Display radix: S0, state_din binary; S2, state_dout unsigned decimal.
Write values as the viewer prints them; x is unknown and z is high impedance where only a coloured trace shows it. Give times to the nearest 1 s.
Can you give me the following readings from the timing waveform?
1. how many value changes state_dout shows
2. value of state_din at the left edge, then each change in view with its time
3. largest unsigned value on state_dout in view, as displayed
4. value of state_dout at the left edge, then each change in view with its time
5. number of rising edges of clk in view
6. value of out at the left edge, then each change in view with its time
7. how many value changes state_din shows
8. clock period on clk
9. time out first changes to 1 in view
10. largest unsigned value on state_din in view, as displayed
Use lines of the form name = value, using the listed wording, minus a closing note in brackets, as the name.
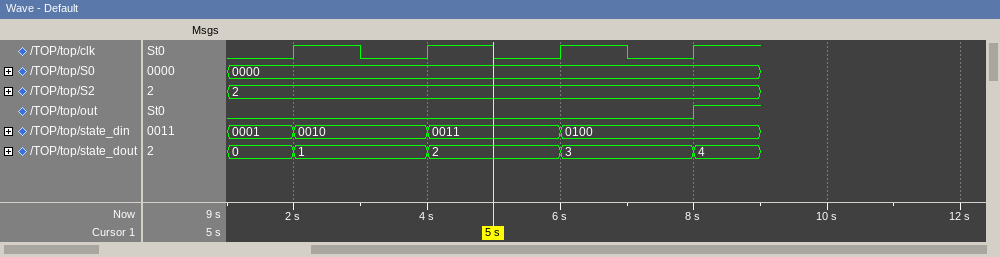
how many value changes state_dout shows = 4
value of state_din at the left edge, then each change in view with its time = 0001, 0010 at 2 s, 0011 at 4 s, 0100 at 6 s
largest unsigned value on state_dout in view, as displayed = 4
value of state_dout at the left edge, then each change in view with its time = 0, 1 at 2 s, 2 at 4 s, 3 at 6 s, 4 at 8 s
number of rising edges of clk in view = 4
value of out at the left edge, then each change in view with its time = 0, 1 at 8 s
how many value changes state_din shows = 3
clock period on clk = 2 s
time out first changes to 1 in view = 8 s
largest unsigned value on state_din in view, as displayed = 0100
